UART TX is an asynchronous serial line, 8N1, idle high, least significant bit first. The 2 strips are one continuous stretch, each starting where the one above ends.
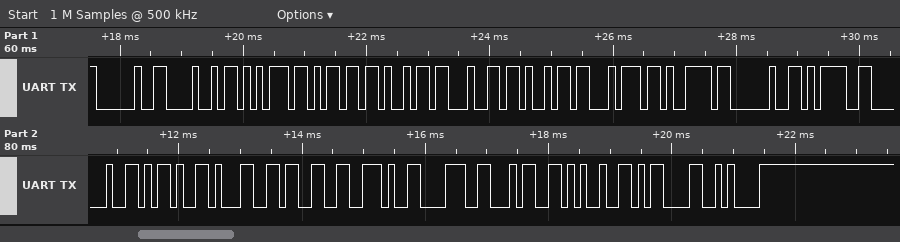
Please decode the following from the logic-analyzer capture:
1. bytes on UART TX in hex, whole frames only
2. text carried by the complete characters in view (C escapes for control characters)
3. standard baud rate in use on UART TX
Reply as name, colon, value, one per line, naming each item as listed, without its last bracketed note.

bytes on UART TX in hex, whole frames only: 0x20 0x48 0x75 0x6D 0x69 0x64 0x69 0x74 0x79 0x20 0x3D 0x20 0x2D 0x31 0x33 0x2E 0x38 0x34 0x25 0x0D 0x0A
text carried by the complete characters in view: " Humidity = -13.84%\r\n"
standard baud rate in use on UART TX: 9600 baud
